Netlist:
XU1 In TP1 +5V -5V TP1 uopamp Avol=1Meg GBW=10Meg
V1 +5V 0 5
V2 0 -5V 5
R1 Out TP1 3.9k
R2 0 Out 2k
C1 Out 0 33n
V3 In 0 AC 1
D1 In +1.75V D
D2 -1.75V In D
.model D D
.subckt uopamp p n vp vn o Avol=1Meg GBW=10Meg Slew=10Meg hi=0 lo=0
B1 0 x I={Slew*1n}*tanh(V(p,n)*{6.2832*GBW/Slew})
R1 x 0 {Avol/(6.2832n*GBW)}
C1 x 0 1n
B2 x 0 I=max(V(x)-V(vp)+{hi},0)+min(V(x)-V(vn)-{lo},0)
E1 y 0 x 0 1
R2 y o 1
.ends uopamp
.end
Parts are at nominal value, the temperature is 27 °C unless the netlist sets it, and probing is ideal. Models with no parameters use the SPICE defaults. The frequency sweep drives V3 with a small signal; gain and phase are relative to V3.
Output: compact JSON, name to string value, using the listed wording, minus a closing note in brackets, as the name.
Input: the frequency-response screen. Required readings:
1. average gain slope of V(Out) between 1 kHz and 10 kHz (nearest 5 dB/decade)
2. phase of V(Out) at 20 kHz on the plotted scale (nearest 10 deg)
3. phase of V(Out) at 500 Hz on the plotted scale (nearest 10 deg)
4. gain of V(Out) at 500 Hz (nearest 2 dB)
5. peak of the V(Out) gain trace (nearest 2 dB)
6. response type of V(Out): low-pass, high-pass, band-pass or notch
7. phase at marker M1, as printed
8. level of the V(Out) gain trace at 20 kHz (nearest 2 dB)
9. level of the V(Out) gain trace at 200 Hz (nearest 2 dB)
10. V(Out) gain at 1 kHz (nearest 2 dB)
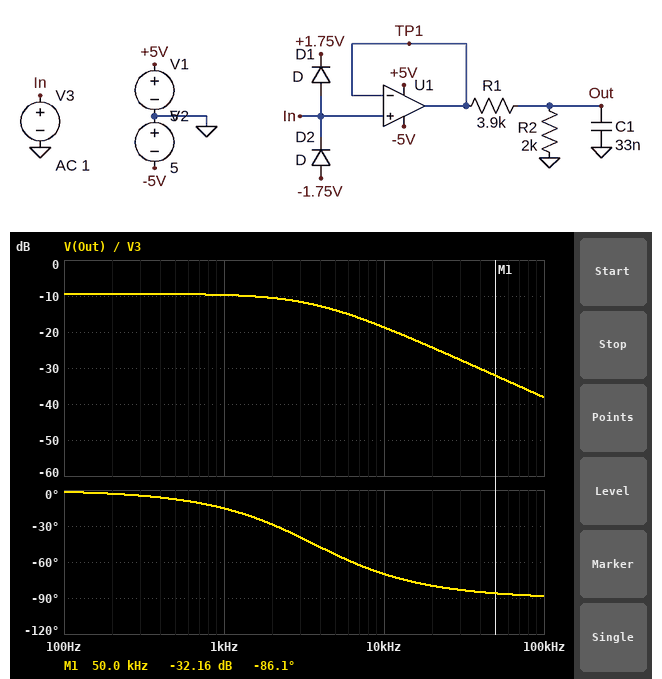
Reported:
{"average gain slope of V(Out) between 1 kHz and 10 kHz": "-10 dB/decade", "phase of V(Out) at 20 kHz on the plotted scale": "-80 deg", "phase of V(Out) at 500 Hz on the plotted scale": "-10 deg", "gain of V(Out) at 500 Hz": "-10 dB", "peak of the V(Out) gain trace": "-10 dB", "response type of V(Out): low-pass, high-pass, band-pass or notch": "low-pass", "phase at marker M1, as printed": "-86.1 deg", "level of the V(Out) gain trace at 20 kHz": "-24 dB", "level of the V(Out) gain trace at 200 Hz": "-10 dB", "V(Out) gain at 1 kHz": "-10 dB"}
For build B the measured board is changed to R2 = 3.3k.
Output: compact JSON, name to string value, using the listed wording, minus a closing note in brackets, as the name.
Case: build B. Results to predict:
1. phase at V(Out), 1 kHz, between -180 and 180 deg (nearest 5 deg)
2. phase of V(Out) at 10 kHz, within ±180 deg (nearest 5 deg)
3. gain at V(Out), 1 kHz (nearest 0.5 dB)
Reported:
{"phase at V(Out), 1 kHz, between -180 and 180 deg": "-20 deg", "phase of V(Out) at 10 kHz, within ±180 deg": "-75 deg", "gain at V(Out), 1 kHz": "-7.5 dB"}
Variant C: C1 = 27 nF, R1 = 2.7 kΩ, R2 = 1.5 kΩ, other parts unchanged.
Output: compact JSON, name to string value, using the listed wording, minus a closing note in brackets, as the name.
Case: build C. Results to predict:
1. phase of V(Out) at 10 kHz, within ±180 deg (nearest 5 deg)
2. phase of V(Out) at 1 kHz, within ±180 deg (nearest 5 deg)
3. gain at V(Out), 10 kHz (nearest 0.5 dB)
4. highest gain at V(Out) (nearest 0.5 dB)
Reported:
{"phase of V(Out) at 10 kHz, within ±180 deg": "-60 deg", "phase of V(Out) at 1 kHz, within ±180 deg": "-10 deg", "gain at V(Out), 10 kHz": "-14.5 dB", "highest gain at V(Out)": "-9.0 dB"}
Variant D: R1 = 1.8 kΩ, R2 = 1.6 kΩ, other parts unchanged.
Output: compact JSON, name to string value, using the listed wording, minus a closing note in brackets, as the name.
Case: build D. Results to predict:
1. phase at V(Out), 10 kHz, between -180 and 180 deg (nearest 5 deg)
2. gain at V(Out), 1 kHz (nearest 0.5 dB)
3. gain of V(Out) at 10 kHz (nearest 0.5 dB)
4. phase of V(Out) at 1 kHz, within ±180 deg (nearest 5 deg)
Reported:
{"phase at V(Out), 10 kHz, between -180 and 180 deg": "-60 deg", "gain at V(Out), 1 kHz": "-6.5 dB", "gain of V(Out) at 10 kHz": "-12.5 dB", "phase of V(Out) at 1 kHz, within ±180 deg": "-10 deg"}
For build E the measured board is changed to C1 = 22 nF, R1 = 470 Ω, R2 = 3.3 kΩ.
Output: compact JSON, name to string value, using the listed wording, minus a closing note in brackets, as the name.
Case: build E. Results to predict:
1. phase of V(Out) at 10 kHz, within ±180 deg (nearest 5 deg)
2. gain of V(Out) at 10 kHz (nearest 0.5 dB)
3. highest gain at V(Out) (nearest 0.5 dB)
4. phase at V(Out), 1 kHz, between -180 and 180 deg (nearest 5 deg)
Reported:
{"phase of V(Out) at 10 kHz, within ±180 deg": "-30 deg", "gain of V(Out) at 10 kHz": "-2.5 dB", "highest gain at V(Out)": "-1.0 dB", "phase at V(Out), 1 kHz, between -180 and 180 deg": "-5 deg"}
